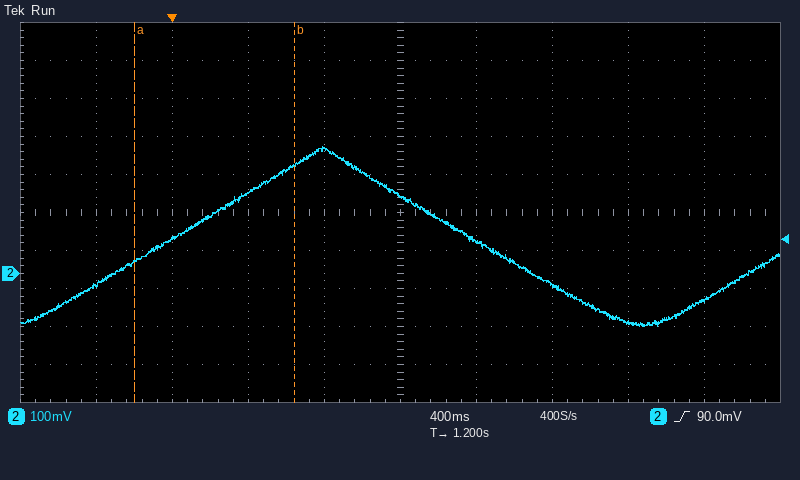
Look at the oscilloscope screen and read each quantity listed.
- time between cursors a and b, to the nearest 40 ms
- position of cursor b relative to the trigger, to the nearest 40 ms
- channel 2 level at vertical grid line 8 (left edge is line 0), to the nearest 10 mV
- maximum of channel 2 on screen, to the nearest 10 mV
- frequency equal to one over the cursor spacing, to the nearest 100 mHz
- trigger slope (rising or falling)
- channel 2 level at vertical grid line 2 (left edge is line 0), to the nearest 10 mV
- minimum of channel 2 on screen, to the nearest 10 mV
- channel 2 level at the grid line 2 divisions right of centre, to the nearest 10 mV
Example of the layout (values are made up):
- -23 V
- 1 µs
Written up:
- 840 ms
- +640 ms
- -130 mV
- 330 mV
- 1.2 Hz
- rising
- 90 mV
- -140 mV
- -30 mV
